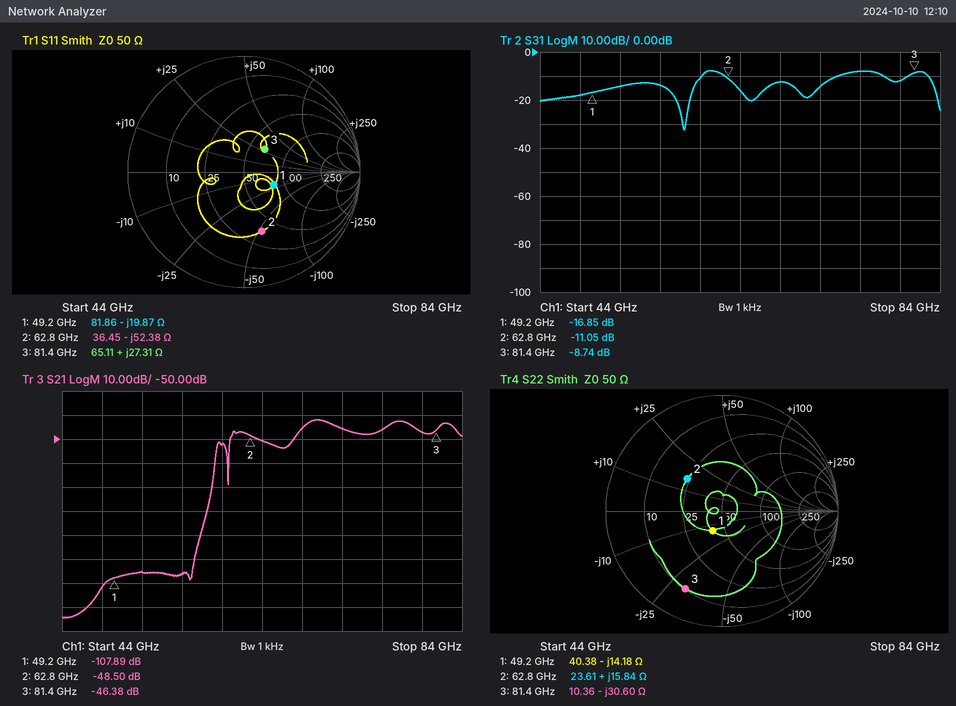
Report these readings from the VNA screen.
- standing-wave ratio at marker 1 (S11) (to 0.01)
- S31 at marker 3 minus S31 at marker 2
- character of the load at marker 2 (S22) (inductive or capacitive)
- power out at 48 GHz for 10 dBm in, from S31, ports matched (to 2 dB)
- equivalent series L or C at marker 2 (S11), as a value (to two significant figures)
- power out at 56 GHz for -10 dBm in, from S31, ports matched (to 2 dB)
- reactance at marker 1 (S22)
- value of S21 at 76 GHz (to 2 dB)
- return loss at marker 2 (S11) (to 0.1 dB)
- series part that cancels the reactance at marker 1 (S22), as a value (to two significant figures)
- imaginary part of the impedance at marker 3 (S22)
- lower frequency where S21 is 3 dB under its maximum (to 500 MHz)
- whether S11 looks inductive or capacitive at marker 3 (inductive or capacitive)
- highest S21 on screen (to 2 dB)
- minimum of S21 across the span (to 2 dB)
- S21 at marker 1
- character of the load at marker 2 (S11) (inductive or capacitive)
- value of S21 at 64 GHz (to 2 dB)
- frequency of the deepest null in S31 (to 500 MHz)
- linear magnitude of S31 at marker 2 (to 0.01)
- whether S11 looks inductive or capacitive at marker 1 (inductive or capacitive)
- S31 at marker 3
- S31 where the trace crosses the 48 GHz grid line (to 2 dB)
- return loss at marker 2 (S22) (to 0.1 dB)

1.78
2.31 dB
inductive
-8 dBm
48 fF
-24 dBm
-14.18 Ω
-46 dB
5.4 dB
46 pH
-30.60 Ω
68.0 GHz
inductive
-42 dB
-124 dB
-107.89 dB
capacitive
-50 dB
58.5 GHz
0.28
capacitive
-8.74 dB
-18 dB
7.8 dB
